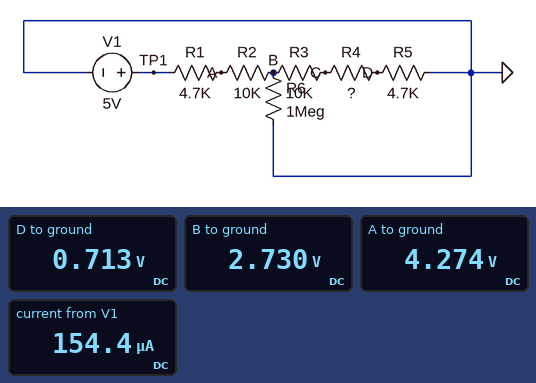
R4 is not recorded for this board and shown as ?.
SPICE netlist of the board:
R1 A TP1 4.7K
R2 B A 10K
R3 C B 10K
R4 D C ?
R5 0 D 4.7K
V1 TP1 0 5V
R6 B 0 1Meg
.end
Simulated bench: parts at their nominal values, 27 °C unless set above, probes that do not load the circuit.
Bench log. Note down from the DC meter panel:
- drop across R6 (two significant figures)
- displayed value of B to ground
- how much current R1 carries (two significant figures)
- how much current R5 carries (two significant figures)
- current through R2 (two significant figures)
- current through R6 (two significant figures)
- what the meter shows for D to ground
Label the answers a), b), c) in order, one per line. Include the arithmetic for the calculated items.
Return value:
a) 2.73 V = 2.7 V
b) 2.730 V
c) (5 V - 4.274 V) / 4.7 kΩ = 150 µA
d) (713 mV) / 4.7 kΩ = 150 µA
e) (4.274 V - 2.73 V) / 10 kΩ = 150 µA
f) (2.73 V) / 1 MΩ = 2.7 µA
g) 0.713 V
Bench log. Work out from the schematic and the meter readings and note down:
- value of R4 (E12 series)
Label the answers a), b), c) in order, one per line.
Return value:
a) 3.3 kΩ
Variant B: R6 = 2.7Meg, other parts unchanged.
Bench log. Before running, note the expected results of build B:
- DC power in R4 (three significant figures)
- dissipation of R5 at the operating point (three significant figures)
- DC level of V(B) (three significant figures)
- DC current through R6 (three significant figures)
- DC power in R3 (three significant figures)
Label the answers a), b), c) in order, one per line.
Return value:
a) 76.7 µW
b) 109 µW
c) 2.74 V
d) 1.02 µA
e) 232 µW
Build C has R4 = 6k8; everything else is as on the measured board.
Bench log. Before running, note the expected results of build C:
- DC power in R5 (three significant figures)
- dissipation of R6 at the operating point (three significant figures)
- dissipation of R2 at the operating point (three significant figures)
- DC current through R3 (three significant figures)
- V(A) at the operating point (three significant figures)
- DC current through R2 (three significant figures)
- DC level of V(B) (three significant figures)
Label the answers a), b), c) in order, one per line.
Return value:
a) 88.1 µW
b) 8.67 µW
c) 196 µW
d) 137 µA
e) 4.34 V
f) 140 µA
g) 2.94 V
